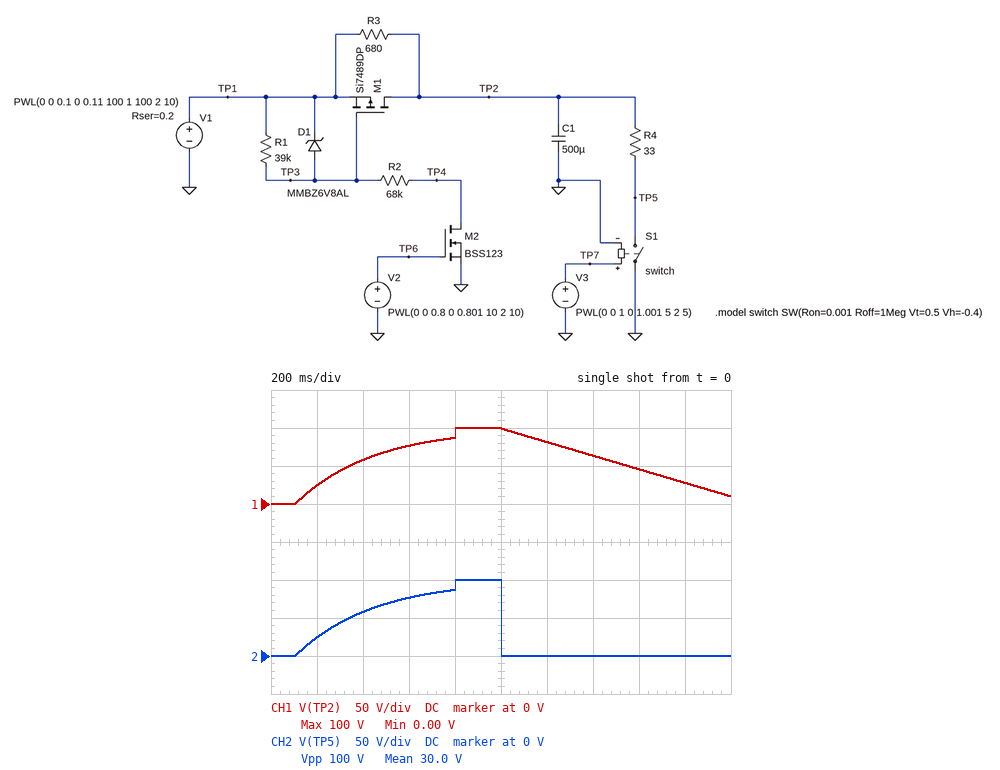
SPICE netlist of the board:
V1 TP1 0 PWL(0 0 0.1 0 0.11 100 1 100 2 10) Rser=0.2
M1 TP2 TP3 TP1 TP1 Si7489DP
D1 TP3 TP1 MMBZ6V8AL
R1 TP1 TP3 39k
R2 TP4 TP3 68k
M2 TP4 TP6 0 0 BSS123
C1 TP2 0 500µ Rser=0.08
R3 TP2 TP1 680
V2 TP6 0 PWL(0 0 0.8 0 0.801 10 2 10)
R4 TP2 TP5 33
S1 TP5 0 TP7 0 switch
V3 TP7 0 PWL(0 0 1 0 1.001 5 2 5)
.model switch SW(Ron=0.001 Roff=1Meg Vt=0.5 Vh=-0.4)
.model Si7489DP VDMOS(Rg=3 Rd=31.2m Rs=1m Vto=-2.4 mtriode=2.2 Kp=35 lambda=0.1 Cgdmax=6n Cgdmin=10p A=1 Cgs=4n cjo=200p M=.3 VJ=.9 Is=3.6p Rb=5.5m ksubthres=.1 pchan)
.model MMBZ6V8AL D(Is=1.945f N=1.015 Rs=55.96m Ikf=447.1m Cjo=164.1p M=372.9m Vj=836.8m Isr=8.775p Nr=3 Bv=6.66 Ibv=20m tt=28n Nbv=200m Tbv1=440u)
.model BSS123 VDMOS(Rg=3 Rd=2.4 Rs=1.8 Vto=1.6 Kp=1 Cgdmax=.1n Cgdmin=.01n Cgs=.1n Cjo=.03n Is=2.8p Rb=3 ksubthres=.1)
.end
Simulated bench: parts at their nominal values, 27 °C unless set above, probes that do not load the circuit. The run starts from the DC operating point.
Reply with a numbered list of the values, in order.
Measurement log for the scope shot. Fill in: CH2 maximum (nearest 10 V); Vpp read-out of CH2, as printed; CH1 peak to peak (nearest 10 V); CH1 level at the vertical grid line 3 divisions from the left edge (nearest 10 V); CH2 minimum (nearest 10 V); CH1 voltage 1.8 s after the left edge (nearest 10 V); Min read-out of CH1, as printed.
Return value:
1. 100 V
2. 100 V
3. 100 V
4. 80 V
5. 0 V
6. 30 V
7. 0.00 V
